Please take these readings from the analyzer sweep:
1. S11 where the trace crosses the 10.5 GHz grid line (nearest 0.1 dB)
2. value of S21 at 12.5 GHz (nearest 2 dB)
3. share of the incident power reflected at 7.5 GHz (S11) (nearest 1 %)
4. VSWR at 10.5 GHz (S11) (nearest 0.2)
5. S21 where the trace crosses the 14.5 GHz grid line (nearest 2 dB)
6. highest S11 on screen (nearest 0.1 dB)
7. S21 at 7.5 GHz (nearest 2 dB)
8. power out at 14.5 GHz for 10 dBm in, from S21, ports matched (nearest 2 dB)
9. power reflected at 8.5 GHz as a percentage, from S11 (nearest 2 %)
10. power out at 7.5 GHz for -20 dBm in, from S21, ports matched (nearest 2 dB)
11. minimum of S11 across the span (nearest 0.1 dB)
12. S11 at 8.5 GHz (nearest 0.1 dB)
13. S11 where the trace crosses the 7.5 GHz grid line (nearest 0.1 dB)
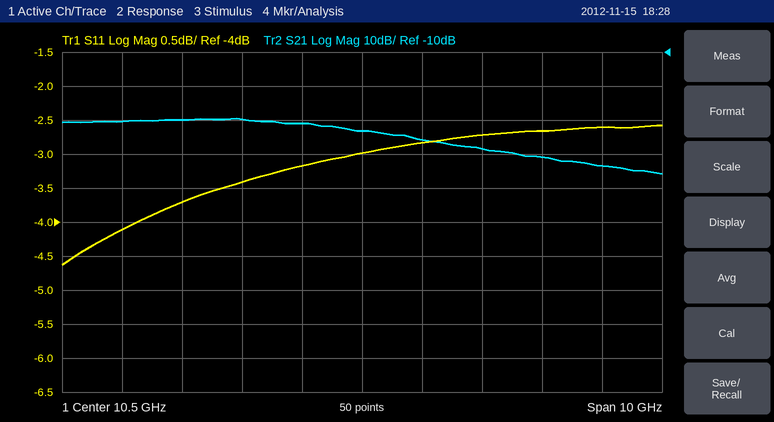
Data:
-3.0 dB
-38 dB
43 %
5.8
-44 dB
-2.6 dB
-30 dB
-34 dBm
46 %
-50 dBm
-4.6 dB
-3.4 dB
-3.7 dB
